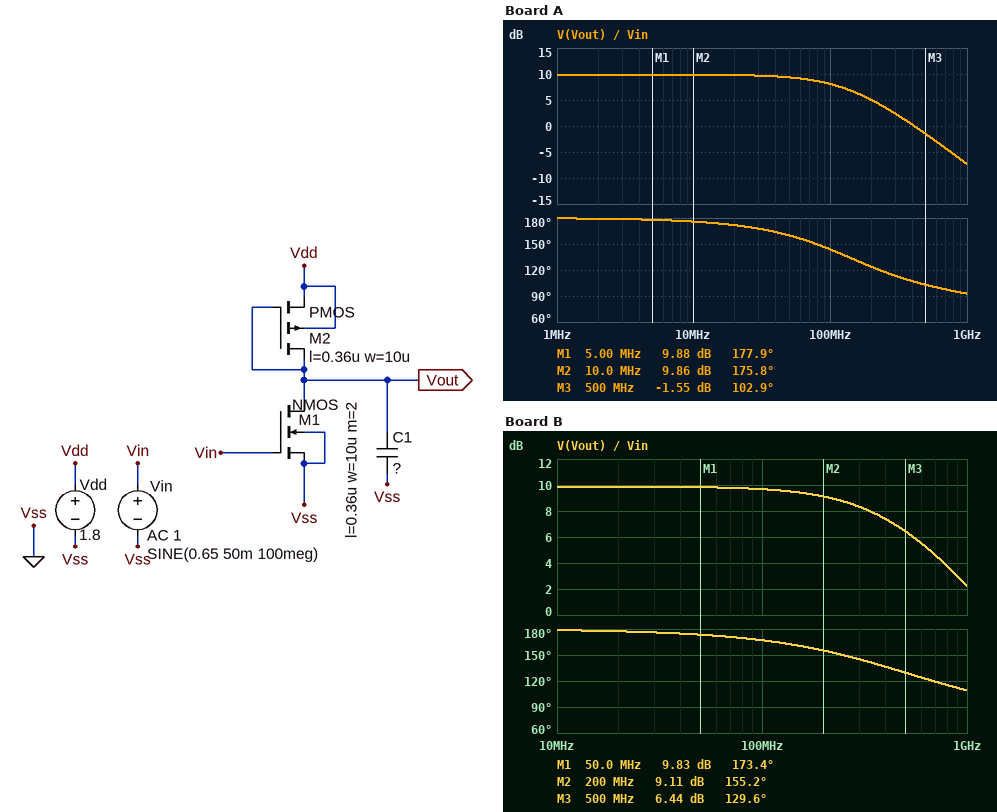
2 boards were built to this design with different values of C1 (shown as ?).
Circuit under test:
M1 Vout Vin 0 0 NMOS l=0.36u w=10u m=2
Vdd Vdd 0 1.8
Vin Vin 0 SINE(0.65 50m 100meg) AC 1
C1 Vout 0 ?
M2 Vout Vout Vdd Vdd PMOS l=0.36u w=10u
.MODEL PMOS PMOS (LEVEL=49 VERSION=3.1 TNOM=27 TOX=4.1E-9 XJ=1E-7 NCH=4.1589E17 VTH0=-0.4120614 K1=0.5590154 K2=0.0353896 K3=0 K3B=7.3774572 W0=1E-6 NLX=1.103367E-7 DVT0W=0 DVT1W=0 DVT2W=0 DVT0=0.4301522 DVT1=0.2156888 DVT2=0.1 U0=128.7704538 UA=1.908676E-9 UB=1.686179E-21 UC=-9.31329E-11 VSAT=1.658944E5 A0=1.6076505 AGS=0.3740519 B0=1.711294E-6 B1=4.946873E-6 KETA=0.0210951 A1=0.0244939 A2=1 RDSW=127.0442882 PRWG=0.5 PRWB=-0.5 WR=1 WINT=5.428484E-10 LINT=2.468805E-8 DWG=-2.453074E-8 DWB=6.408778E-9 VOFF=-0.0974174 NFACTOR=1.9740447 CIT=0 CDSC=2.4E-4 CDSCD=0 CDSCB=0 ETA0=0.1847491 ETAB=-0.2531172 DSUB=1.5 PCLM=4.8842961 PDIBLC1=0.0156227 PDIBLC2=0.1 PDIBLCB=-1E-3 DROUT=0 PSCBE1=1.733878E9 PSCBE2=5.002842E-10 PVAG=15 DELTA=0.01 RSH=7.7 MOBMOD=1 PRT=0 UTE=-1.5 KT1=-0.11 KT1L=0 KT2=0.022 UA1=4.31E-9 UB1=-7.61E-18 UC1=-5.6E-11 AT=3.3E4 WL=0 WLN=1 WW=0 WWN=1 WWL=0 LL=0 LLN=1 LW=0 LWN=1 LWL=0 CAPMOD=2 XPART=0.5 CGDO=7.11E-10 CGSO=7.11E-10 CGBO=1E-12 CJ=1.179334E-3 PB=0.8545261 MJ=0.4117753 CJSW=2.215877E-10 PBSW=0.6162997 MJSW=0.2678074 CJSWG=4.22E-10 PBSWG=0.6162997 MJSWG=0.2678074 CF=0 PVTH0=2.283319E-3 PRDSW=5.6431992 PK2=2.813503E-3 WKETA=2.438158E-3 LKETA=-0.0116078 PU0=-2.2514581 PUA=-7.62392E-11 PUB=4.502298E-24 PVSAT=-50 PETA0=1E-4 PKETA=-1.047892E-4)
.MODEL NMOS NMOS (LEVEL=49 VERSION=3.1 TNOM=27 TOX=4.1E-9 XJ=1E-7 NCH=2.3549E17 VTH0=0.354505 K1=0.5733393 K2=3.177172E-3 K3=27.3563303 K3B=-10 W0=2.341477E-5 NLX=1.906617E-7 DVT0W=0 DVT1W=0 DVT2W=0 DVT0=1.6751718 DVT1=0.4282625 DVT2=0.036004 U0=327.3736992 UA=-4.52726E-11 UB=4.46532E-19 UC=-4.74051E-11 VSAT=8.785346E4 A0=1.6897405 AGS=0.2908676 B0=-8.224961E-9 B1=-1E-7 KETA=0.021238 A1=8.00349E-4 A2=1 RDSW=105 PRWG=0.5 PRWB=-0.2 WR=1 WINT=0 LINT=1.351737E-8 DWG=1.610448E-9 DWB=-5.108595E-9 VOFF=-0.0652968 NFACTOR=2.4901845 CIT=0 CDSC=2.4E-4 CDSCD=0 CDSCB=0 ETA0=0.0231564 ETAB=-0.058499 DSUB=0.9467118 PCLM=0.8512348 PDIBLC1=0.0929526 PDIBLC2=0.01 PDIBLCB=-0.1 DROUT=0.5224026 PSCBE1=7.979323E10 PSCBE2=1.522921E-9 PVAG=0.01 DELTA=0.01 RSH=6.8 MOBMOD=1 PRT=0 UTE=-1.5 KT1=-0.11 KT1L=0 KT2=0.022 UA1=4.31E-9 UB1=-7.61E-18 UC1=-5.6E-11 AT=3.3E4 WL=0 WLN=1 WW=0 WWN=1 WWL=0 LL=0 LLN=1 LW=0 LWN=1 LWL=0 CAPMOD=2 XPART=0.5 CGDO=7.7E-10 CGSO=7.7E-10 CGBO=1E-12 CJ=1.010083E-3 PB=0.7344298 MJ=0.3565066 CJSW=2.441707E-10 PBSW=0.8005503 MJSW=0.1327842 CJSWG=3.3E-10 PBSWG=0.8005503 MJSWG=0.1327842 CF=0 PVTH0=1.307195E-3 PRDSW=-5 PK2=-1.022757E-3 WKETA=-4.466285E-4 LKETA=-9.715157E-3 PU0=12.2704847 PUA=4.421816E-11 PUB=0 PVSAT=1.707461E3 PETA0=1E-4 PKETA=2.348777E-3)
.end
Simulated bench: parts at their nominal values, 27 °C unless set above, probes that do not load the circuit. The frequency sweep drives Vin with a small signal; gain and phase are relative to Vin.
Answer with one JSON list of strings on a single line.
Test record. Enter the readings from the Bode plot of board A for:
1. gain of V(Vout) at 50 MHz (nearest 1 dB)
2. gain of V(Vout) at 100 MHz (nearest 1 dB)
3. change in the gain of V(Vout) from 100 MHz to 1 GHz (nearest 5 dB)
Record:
["9 dB", "8 dB", "-15 dB"]
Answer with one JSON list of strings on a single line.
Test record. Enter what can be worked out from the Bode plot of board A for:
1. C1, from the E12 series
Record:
["820 fF"]
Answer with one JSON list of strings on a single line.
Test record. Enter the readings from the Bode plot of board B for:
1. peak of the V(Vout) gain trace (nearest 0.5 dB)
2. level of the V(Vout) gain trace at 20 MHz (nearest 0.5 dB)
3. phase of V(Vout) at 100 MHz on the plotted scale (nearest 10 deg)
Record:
["10.0 dB", "10.0 dB", "170 deg"]
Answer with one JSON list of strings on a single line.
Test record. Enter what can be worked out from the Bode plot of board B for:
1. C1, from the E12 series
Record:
["220 fF"]
